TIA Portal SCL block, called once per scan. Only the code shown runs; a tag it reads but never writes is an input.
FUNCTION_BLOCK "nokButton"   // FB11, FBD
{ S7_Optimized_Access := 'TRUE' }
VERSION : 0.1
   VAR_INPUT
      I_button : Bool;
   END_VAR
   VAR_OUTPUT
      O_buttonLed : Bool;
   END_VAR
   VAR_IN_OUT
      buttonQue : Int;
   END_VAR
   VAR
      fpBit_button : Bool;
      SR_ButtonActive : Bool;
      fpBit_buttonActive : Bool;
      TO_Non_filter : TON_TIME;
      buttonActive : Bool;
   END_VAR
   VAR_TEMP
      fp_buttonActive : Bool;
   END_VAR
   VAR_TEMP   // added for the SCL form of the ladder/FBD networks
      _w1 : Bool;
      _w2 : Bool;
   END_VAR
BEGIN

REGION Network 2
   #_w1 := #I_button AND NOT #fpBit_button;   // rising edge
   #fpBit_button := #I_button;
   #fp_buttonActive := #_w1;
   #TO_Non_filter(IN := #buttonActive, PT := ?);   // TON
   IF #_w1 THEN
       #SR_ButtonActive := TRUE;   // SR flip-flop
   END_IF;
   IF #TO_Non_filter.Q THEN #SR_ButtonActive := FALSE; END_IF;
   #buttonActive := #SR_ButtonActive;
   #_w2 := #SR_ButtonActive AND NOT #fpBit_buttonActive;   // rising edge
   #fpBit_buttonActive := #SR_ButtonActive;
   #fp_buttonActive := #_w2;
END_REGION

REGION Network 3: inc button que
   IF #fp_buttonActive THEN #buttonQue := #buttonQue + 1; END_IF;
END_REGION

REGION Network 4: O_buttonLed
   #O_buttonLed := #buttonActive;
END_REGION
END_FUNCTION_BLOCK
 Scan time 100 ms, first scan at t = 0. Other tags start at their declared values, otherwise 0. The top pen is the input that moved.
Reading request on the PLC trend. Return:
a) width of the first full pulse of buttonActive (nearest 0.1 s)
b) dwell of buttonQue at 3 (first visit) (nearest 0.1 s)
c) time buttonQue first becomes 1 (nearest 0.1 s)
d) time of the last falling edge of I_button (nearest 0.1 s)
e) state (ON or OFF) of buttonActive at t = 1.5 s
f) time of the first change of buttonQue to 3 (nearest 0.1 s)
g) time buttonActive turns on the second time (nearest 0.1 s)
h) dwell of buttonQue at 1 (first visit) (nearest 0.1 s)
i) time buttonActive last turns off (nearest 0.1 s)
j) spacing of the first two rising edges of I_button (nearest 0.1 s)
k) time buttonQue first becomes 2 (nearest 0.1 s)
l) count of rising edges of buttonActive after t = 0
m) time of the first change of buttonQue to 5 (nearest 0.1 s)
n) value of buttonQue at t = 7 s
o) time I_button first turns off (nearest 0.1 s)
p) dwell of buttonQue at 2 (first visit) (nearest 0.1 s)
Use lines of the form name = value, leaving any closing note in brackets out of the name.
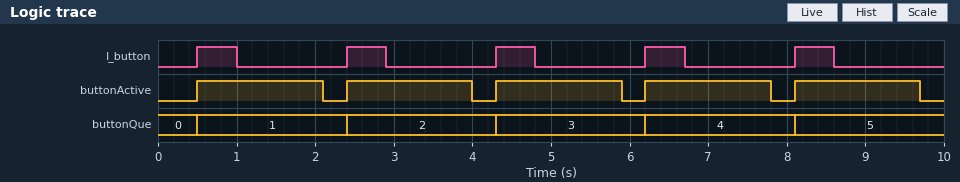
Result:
width of the first full pulse of buttonActive = 1.6 s
dwell of buttonQue at 3 (first visit) = 1.9 s
time buttonQue first becomes 1 = 0.5 s
time of the last falling edge of I_button = 8.6 s
state (ON or OFF) of buttonActive at t = 1.5 s = ON
time of the first change of buttonQue to 3 = 4.3 s
time buttonActive turns on the second time = 2.4 s
dwell of buttonQue at 1 (first visit) = 1.9 s
time buttonActive last turns off = 9.7 s
spacing of the first two rising edges of I_button = 1.9 s
time buttonQue first becomes 2 = 2.4 s
count of rising edges of buttonActive after t = 0 = 5
time of the first change of buttonQue to 5 = 8.1 s
value of buttonQue at t = 7 s = 4
time I_button first turns off = 1.0 s
dwell of buttonQue at 2 (first visit) = 1.9 s
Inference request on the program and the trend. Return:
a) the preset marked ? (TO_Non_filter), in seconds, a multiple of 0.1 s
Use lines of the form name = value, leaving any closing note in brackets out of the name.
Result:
the preset marked ? (TO_Non_filter), in seconds, a multiple of 0.1 s = 1.5 s
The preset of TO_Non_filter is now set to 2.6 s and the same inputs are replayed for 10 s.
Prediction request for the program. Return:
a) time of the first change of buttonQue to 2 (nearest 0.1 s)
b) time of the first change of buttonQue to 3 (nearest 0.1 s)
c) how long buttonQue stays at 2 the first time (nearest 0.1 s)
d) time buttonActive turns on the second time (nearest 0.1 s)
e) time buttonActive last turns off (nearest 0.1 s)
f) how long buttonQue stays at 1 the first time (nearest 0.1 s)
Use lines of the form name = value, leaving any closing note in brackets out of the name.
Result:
time of the first change of buttonQue to 2 = 4.3 s
time of the first change of buttonQue to 3 = 8.1 s
how long buttonQue stays at 2 the first time = 3.8 s
time buttonActive turns on the second time = 4.3 s
time buttonActive last turns off = 7.0 s
how long buttonQue stays at 1 the first time = 3.8 s
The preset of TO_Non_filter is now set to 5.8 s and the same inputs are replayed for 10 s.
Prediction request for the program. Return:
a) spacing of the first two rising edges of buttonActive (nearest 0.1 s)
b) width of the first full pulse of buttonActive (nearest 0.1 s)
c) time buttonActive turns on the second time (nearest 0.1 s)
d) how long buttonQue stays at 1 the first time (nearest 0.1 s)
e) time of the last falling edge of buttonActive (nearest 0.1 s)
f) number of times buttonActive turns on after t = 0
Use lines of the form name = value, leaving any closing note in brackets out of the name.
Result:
spacing of the first two rising edges of buttonActive = 7.6 s
width of the first full pulse of buttonActive = 5.9 s
time buttonActive turns on the second time = 8.1 s
how long buttonQue stays at 1 the first time = 7.6 s
time of the last falling edge of buttonActive = 6.4 s
number of times buttonActive turns on after t = 0 = 2
